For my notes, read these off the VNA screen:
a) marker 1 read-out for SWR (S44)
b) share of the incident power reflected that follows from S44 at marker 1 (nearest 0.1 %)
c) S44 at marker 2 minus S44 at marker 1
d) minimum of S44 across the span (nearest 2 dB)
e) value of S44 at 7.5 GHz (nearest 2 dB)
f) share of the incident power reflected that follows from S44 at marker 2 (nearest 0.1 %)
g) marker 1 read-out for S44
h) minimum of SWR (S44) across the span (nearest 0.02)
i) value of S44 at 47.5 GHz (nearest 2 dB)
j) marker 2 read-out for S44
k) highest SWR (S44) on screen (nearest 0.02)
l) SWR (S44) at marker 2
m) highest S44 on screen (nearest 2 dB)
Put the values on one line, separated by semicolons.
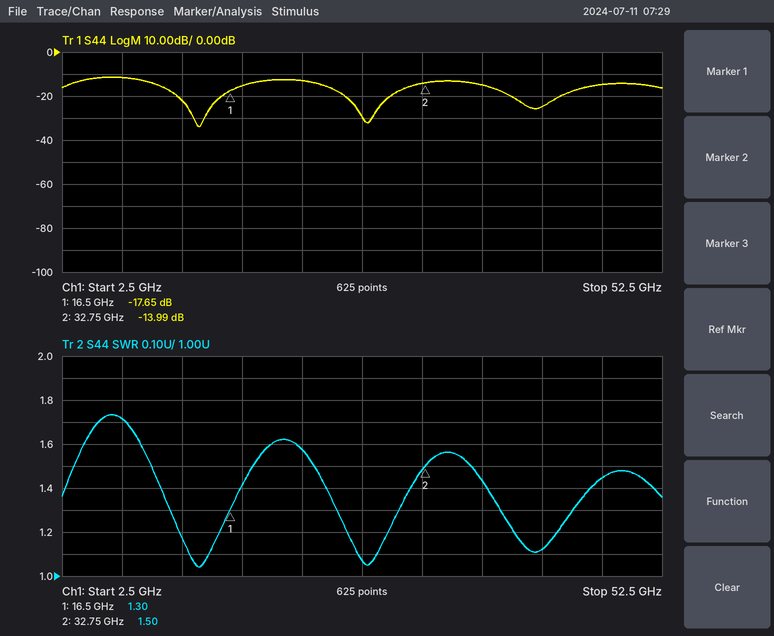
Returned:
1.30; 1.7 %; 3.66 dB; -34 dB; -12 dB; 4.0 %; -17.65 dB; 1.04; -14 dB; -13.99 dB; 1.74; 1.50; -12 dB
